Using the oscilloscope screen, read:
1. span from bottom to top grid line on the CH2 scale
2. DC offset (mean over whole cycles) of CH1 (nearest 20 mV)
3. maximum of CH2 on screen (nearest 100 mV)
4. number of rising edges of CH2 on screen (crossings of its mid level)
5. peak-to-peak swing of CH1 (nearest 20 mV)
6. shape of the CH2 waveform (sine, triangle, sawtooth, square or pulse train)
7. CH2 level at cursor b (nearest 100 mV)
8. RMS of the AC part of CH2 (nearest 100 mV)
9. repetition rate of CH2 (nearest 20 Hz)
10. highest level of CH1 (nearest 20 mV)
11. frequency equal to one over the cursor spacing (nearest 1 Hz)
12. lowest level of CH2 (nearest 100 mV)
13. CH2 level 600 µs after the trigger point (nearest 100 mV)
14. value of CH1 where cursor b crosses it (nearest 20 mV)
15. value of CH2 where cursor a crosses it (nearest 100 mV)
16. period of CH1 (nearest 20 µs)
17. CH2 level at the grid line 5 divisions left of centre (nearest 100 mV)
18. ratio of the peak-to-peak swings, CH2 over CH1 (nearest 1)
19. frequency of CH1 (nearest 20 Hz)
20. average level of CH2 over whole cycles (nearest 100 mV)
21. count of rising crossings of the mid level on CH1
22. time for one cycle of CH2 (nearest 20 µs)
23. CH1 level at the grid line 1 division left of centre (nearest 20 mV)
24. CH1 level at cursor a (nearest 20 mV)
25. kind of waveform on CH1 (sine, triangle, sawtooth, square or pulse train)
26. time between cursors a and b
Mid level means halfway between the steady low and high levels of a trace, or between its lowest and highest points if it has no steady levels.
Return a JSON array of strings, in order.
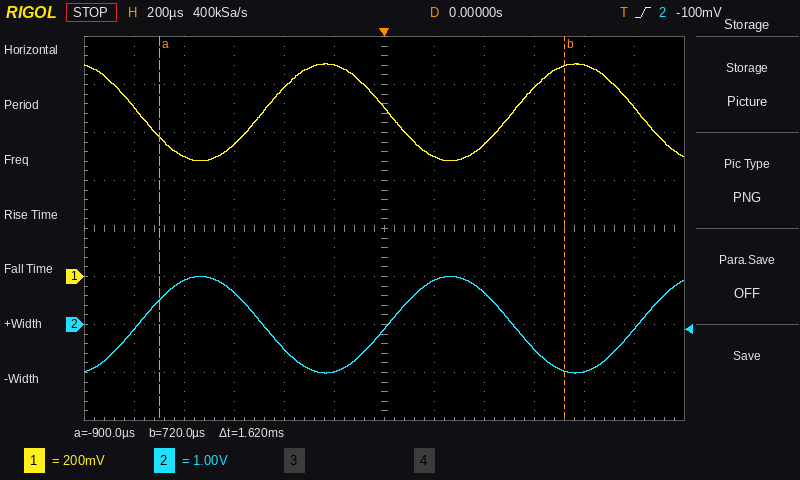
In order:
["8 V", "680 mV", "1.0 V", "3", "400 mV", "sine", "-1.0 V", "700 mV", "1.00 kHz", "880 mV", "617 Hz", "-1.0 V", "-500 mV", "880 mV", "500 mV", "1.00 ms", "-100 mV", "5", "1.00 kHz", "0.0 V", "2", "1.00 ms", "880 mV", "580 mV", "sine", "1.62 ms"]
